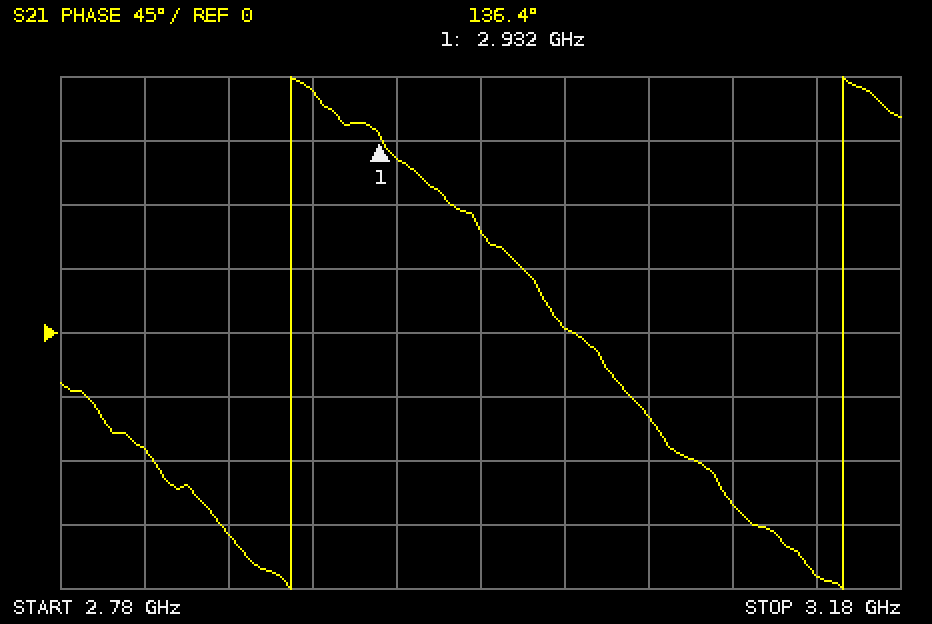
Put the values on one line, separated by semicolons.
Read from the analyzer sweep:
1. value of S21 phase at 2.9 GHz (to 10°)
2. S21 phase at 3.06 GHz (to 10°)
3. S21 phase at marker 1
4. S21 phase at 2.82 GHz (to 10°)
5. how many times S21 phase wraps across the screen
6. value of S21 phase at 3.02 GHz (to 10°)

170°; -60°; 136.4°; -80°; 2; 0°
